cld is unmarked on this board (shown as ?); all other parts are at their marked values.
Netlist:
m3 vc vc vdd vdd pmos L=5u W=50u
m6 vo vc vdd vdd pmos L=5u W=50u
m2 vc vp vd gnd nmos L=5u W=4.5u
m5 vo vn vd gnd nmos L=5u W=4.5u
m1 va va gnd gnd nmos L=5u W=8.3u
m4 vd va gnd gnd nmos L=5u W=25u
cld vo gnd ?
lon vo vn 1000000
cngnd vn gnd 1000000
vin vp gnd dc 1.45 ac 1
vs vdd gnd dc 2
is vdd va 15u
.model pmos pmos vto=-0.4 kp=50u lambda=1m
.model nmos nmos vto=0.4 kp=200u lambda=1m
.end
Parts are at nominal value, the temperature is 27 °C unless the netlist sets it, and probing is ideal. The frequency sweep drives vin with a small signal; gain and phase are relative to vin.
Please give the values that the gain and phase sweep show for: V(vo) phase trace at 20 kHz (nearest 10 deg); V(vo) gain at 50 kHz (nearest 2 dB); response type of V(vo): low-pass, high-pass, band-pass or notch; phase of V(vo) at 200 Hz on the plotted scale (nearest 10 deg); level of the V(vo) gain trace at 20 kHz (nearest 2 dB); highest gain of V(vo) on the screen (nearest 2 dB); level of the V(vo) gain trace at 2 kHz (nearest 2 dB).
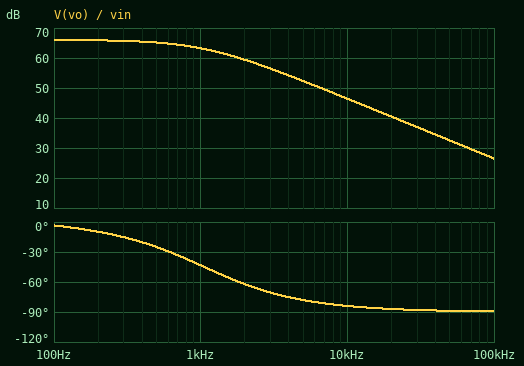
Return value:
-90 deg
32 dB
low-pass
-10 deg
40 dB
66 dB
60 dB
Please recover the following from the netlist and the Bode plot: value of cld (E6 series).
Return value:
6.8 pF
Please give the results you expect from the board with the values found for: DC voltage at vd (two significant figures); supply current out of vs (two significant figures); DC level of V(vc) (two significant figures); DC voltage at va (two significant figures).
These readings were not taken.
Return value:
550 mV
60 µA
1.3 V
700 mV
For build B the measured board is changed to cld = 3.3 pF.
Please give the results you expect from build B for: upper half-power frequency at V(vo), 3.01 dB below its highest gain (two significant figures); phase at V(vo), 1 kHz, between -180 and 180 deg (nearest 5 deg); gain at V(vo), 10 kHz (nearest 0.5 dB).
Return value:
2.2 kHz
-25 deg
52.5 dB
